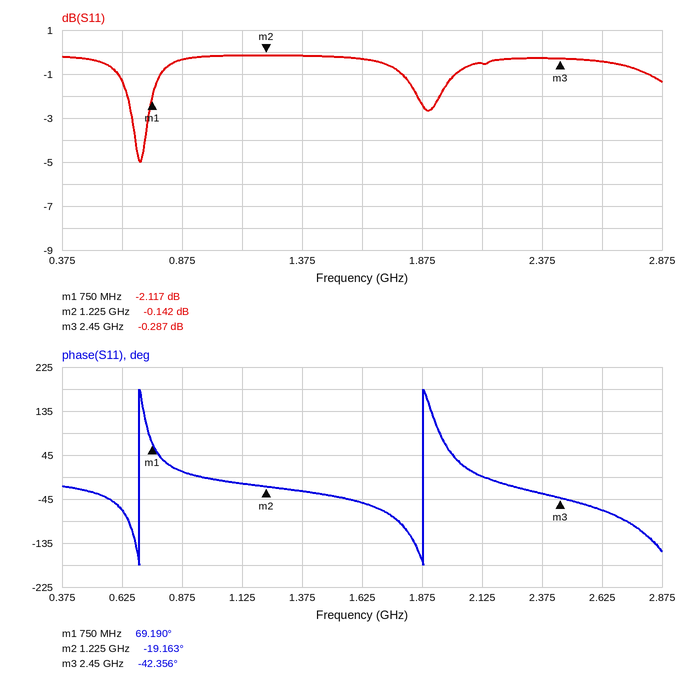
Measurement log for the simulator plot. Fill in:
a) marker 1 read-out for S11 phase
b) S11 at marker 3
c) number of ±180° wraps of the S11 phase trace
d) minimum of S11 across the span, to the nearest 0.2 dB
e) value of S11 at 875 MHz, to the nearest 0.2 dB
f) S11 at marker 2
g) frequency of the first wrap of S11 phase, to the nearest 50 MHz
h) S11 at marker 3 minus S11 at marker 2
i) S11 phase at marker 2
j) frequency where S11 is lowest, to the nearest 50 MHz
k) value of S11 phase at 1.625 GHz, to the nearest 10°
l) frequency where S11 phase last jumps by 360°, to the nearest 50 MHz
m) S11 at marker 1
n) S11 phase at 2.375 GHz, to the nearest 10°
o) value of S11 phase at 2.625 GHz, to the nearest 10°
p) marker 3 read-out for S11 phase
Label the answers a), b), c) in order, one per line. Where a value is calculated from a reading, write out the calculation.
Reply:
a) 69.190°
b) -0.287 dB
c) 2
d) -5.0 dB
e) -0.4 dB
f) -0.142 dB
g) 700 MHz
h) -0.287 − (-0.142) = -0.145 dB
i) -19.163°
j) 700 MHz
k) -50°
l) 1.90 GHz
m) -2.117 dB
n) -30°
o) -70°
p) -42.356°
